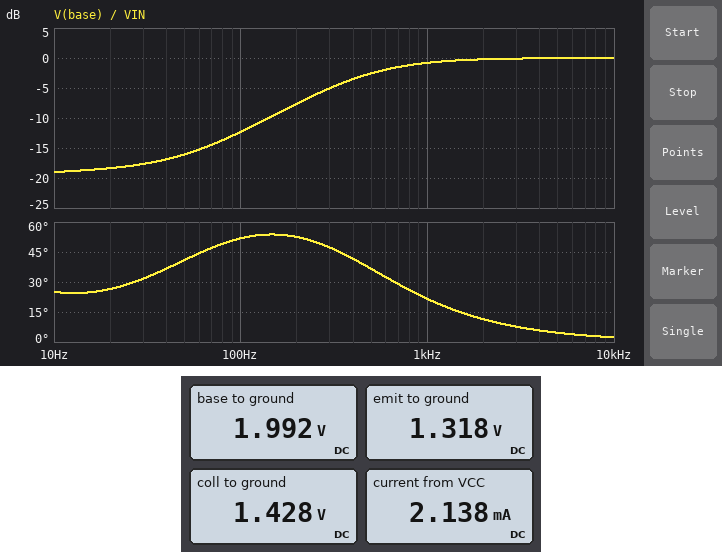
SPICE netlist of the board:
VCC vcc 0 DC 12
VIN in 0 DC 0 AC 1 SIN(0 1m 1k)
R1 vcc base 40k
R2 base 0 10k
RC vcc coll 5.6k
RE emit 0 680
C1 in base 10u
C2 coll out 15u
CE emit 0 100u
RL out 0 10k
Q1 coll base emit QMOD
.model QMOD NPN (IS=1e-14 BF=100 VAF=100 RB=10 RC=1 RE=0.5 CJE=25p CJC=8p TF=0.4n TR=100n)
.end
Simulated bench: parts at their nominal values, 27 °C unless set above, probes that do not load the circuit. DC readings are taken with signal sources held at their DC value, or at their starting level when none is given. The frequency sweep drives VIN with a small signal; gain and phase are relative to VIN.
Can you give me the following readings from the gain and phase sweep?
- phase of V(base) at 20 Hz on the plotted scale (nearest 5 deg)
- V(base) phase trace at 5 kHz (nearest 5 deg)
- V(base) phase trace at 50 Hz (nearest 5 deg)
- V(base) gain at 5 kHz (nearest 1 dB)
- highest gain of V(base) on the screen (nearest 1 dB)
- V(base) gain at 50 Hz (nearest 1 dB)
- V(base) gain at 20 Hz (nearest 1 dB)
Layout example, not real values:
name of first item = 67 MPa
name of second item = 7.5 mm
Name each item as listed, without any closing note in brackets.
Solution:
phase of V(base) at 20 Hz on the plotted scale = 25 deg
V(base) phase trace at 5 kHz = 5 deg
V(base) phase trace at 50 Hz = 40 deg
V(base) gain at 5 kHz = 0 dB
highest gain of V(base) on the screen = 0 dB
V(base) gain at 50 Hz = -16 dB
V(base) gain at 20 Hz = -18 dB
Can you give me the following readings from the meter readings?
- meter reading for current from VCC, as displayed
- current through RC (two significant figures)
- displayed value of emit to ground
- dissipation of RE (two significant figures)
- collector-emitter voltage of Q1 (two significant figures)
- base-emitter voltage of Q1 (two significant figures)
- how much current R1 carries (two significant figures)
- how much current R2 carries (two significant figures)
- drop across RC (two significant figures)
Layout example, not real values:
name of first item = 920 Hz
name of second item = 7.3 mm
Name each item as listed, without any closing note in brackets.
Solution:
meter reading for current from VCC, as displayed = 2.138 mA
current through RC = 1.9 mA
displayed value of emit to ground = 1.318 V
dissipation of RE = 2.6 mW
collector-emitter voltage of Q1 = 110 mV
base-emitter voltage of Q1 = 670 mV
how much current R1 carries = 250 µA
how much current R2 carries = 200 µA
drop across RC = 11 V
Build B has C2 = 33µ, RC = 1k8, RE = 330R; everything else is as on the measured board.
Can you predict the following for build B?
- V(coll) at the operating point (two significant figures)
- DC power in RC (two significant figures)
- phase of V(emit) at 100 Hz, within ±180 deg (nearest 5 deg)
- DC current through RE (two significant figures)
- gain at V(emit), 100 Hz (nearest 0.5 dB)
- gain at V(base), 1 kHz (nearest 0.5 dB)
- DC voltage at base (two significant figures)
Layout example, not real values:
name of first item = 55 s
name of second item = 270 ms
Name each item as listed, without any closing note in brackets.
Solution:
V(coll) at the operating point = 4.5 V
DC power in RC = 31 mW
phase of V(emit) at 100 Hz, within ±180 deg = -20 deg
DC current through RE = 4.2 mA
gain at V(emit), 100 Hz = -1.5 dB
gain at V(base), 1 kHz = 0 dB
DC voltage at base = 2.1 V
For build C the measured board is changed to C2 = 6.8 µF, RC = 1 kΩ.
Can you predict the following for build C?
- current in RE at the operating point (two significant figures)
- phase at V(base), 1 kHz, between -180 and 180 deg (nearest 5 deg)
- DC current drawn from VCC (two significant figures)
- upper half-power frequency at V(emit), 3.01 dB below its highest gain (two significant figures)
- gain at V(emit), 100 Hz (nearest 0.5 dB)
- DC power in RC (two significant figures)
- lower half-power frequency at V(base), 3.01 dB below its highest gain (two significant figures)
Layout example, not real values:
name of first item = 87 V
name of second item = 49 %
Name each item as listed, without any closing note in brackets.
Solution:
current in RE at the operating point = 2.3 mA
phase at V(base), 1 kHz, between -180 and 180 deg = 0 deg
DC current drawn from VCC = 2.5 mA
upper half-power frequency at V(emit), 3.01 dB below its highest gain = 150 Hz
gain at V(emit), 100 Hz = -2.5 dB
DC power in RC = 5.1 mW
lower half-power frequency at V(base), 3.01 dB below its highest gain = 2.5 Hz
